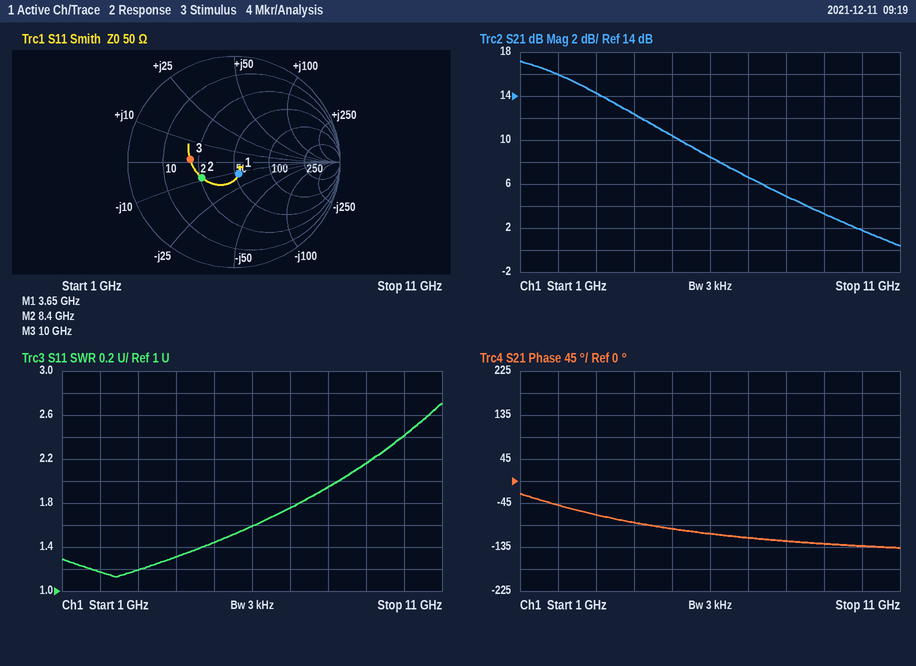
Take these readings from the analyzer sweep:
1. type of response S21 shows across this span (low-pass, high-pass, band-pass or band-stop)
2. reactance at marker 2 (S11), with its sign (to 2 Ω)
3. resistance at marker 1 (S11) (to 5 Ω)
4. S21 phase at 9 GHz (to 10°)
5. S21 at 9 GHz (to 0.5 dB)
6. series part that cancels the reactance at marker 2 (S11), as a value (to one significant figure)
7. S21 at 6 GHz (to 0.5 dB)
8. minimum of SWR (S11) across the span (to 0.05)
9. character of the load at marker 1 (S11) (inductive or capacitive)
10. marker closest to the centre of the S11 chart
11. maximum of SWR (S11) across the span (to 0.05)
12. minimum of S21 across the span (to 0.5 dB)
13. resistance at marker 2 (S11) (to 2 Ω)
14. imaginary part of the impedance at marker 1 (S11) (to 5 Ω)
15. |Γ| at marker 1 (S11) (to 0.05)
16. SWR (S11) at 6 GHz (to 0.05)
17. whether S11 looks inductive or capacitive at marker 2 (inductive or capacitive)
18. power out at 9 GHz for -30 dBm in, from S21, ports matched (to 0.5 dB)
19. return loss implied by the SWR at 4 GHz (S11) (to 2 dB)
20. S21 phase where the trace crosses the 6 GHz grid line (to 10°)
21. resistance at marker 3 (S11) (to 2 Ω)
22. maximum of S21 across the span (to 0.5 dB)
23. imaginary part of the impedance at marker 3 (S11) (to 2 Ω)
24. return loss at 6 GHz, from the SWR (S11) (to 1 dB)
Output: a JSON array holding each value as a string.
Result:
["low-pass", "-8 Ω", "55 Ω", "-130°", "3.5 dB", "200 pH", "8.5 dB", "1.15", "capacitive", "marker 1", "2.70", "0.5 dB", "26 Ω", "-10 Ω", "0.10", "1.60", "capacitive", "-26.5 dBm", "18 dB", "-110°", "20 Ω", "17.0 dB", "+2 Ω", "13 dB"]
